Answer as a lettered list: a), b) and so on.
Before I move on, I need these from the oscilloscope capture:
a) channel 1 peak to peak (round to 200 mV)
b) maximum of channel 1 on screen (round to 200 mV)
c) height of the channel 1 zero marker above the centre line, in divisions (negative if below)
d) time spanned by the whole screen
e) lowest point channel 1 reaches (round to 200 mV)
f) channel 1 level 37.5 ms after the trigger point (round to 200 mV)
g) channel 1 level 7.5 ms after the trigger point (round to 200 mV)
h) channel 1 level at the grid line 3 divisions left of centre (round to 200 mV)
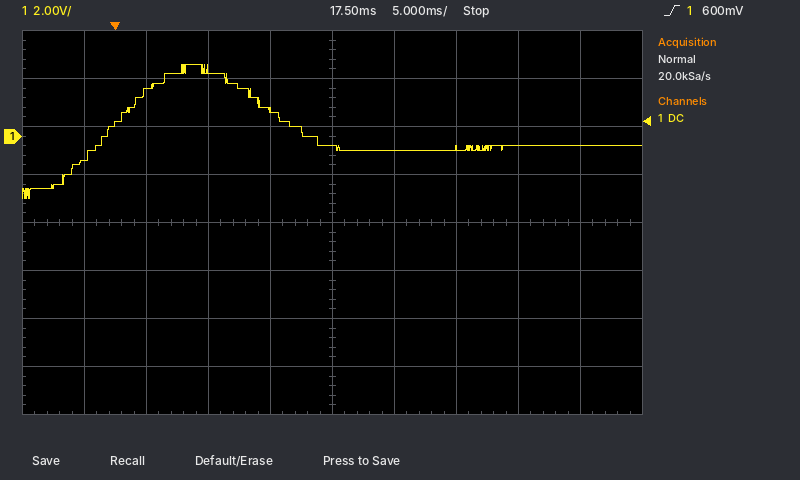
a) 5.6 V
b) 3.0 V
c) +1.8 div
d) 50 ms
e) -2.6 V
f) -400 mV
g) 2.8 V
h) 1.8 V
